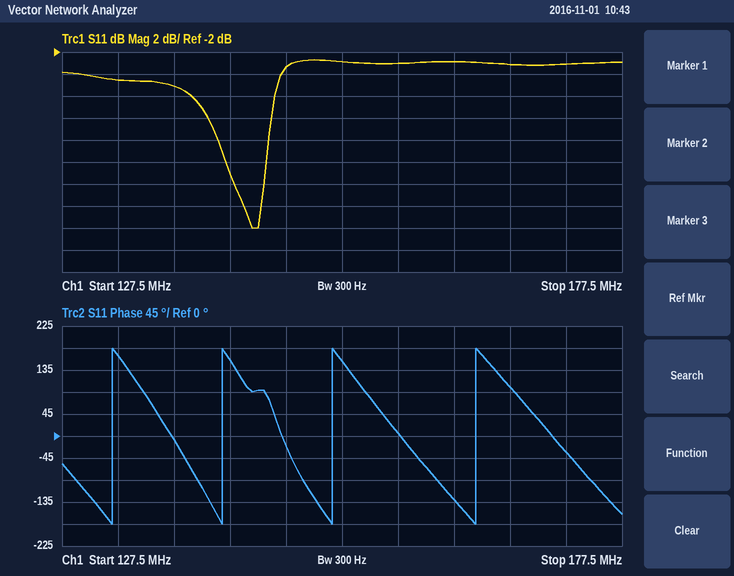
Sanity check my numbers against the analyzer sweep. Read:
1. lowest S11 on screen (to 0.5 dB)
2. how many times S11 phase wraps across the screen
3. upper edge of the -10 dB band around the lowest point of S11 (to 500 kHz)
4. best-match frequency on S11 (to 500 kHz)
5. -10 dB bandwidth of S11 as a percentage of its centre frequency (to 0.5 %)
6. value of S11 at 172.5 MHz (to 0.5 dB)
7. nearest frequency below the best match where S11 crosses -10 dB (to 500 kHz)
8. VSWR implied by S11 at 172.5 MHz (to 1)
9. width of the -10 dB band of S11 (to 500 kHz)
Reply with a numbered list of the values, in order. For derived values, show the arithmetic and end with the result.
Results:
1. -18.0 dB
2. 4
3. 146.0 MHz
4. 144.5 MHz
5. 4.5 MHz / 143.75 MHz ≈ 3.13 %, so 3.0 % to the nearest 0.5 %
6. -3.0 dB
7. 141.5 MHz
8. |Γ| = 10^(-3/20) = 0.7079; VSWR = (1 + 0.7079)/(1 − 0.7079) ≈ 6
9. 146.0 MHz − 141.5 MHz = 4.5 MHz
